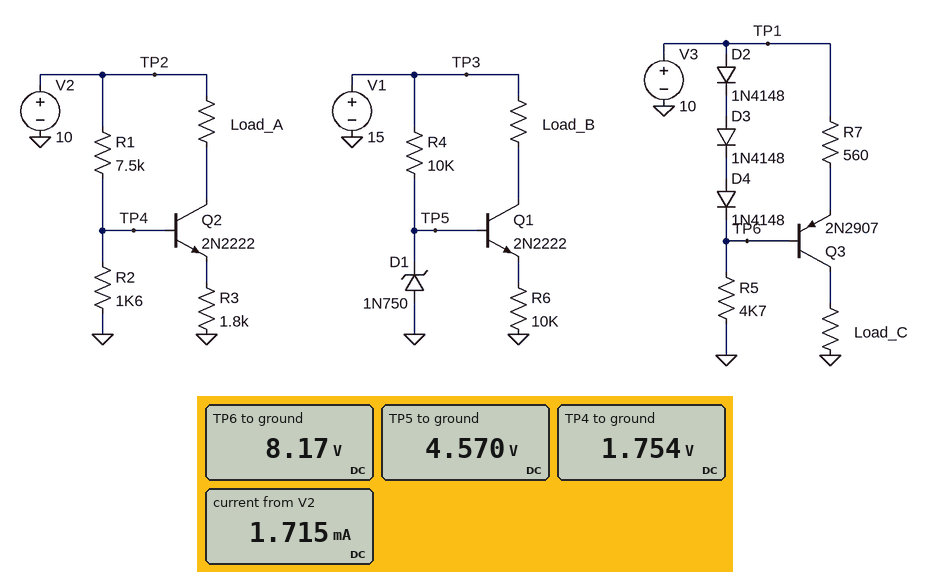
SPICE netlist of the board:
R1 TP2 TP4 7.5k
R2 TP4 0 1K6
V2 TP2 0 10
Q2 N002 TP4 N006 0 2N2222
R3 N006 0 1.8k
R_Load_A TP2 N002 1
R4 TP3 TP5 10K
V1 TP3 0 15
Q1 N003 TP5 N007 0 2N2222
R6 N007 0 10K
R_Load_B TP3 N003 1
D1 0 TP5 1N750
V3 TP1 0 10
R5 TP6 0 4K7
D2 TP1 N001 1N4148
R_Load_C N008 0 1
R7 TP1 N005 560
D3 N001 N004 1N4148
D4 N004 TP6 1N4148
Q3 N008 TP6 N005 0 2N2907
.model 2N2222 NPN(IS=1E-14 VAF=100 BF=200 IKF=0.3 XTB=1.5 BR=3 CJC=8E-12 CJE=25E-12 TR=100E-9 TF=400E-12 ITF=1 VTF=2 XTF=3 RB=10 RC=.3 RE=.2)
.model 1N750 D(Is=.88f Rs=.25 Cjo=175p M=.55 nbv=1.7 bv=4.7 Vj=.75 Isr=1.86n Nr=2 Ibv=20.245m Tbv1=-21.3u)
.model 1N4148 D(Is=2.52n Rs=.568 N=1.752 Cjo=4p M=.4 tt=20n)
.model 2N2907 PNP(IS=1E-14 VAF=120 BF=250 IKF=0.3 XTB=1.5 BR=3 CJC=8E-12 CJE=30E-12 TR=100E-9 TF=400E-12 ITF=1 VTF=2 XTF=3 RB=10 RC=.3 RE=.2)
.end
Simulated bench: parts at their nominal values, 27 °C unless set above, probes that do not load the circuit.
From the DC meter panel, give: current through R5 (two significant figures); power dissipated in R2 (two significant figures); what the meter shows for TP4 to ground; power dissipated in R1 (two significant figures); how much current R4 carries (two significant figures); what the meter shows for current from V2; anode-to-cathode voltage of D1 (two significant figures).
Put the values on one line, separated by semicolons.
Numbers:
1.7 mA; 1.9 mW; 1.754 V; 9.1 mW; 1.0 mA; 1.715 mA; -4.6 V
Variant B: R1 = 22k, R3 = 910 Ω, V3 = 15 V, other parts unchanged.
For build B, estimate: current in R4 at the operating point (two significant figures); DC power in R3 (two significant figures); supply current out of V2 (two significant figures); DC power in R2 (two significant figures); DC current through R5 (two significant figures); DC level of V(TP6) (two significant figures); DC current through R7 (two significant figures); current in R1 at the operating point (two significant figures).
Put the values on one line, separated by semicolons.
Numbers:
1.0 mA; 8.1 µW; 520 µA; 290 µW; 2.8 mA; 13 V; 2.2 mA; 420 µA
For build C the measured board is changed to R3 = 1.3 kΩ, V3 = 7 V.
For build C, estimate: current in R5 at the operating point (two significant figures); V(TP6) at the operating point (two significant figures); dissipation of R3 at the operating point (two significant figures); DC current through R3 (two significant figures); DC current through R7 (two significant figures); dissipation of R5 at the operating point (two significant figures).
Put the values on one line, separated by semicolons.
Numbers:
1.1 mA; 5.2 V; 940 µW; 850 µA; 2.0 mA; 5.8 mW
